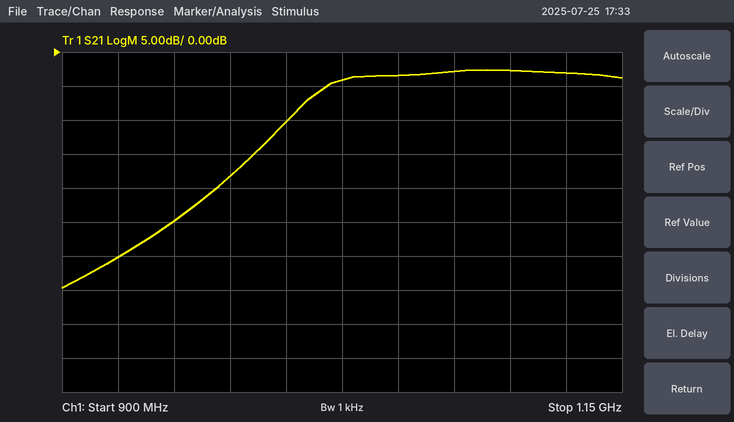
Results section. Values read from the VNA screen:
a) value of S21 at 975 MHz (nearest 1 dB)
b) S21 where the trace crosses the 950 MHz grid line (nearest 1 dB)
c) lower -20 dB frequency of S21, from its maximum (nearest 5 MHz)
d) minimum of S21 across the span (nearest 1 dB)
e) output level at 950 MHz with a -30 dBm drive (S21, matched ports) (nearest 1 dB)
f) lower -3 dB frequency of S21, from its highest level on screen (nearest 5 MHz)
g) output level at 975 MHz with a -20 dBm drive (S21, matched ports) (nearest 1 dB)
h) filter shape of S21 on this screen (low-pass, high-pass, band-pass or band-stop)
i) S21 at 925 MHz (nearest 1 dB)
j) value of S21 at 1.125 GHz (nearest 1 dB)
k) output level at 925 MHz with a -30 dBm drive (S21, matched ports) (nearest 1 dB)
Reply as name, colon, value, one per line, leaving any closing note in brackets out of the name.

value of S21 at 975 MHz: -18 dB
S21 where the trace crosses the 950 MHz grid line: -25 dB
lower -20 dB frequency of S21, from its maximum: 960 MHz
minimum of S21 across the span: -35 dB
output level at 950 MHz with a -30 dBm drive (S21, matched ports): -55 dBm
lower -3 dB frequency of S21, from its highest level on screen: 1.015 GHz
output level at 975 MHz with a -20 dBm drive (S21, matched ports): -38 dBm
filter shape of S21 on this screen: high-pass
S21 at 925 MHz: -30 dB
value of S21 at 1.125 GHz: -3 dB
output level at 925 MHz with a -30 dBm drive (S21, matched ports): -60 dBm
